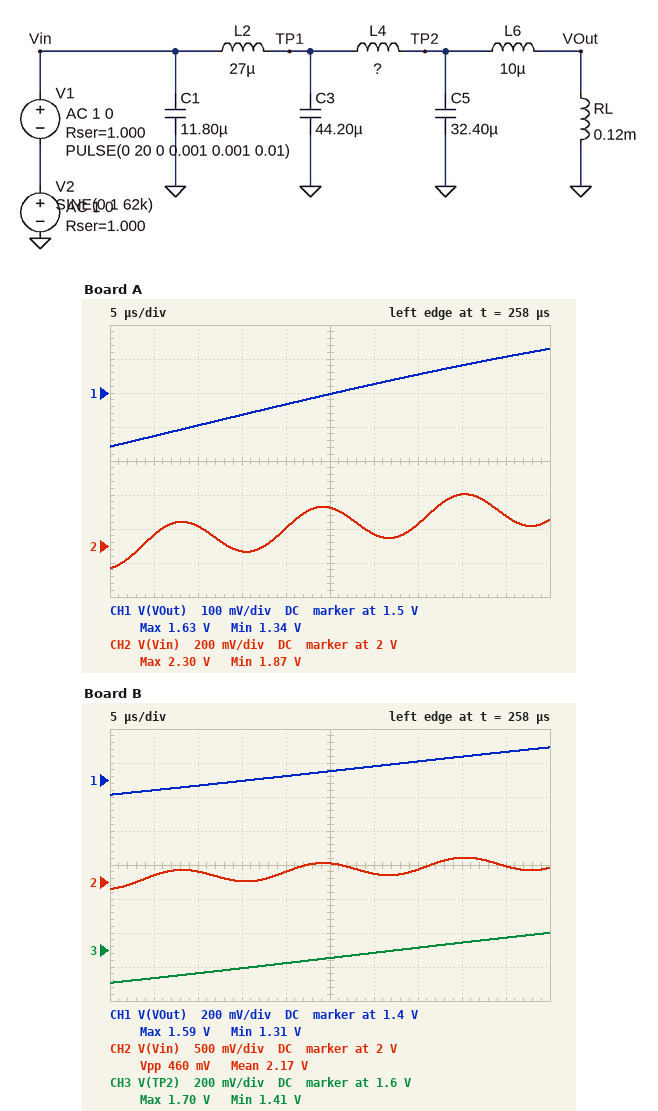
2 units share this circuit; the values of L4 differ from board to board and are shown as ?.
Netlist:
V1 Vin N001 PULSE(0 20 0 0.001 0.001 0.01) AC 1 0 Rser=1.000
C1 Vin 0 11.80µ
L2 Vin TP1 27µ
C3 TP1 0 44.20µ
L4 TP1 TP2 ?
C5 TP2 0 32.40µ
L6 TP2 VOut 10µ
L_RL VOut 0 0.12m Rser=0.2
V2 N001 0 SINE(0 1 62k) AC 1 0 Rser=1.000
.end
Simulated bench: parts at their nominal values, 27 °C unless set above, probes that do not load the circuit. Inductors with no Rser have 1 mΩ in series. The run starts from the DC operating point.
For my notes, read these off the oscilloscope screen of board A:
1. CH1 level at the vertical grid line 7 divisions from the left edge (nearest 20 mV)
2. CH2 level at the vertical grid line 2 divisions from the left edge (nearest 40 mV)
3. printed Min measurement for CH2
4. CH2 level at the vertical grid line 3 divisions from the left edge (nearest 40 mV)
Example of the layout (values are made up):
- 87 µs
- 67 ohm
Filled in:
- 1.56 V
- 2.12 V
- 1.87 V
- 1.96 V
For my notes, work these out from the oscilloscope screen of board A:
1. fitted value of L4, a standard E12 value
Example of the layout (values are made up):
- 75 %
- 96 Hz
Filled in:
- 33 µH
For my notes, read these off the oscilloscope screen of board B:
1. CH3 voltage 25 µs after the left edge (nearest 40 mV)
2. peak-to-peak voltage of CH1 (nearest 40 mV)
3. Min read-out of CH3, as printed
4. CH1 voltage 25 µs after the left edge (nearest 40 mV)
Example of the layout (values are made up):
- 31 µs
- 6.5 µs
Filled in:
- 1.56 V
- 280 mV
- 1.41 V
- 1.44 V
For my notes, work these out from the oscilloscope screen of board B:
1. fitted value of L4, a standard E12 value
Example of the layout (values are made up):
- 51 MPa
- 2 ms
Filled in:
- 39 µH
